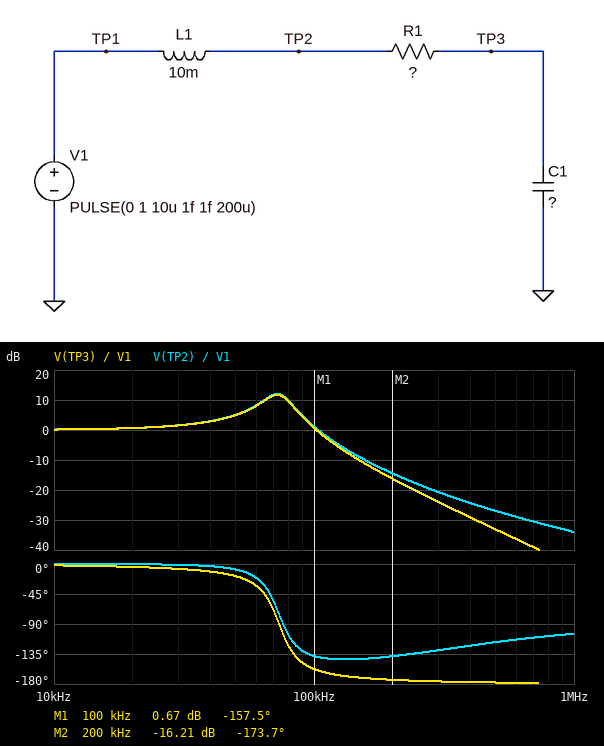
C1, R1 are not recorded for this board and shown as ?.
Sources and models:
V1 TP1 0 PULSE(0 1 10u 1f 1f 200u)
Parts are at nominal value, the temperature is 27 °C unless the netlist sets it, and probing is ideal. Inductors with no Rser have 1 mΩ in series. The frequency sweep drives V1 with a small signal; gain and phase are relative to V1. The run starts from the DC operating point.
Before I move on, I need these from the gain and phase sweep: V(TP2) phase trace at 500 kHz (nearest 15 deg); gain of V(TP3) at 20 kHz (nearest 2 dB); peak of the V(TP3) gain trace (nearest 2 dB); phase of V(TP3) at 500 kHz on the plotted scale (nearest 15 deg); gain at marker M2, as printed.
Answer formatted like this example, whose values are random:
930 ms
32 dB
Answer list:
-120 deg
0 dB
12 dB
-180 deg
-16.21 dB
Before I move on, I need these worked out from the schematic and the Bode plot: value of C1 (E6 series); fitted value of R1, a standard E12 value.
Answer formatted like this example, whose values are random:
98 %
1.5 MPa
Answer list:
470 pF
1.2 kΩ
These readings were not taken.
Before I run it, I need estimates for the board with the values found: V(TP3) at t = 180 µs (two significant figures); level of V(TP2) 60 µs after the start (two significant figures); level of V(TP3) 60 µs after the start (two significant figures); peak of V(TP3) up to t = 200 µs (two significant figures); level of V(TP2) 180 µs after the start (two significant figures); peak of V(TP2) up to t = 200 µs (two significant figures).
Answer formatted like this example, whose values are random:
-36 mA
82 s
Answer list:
1.0 V
1.0 V
1.0 V
1.7 V
1.0 V
1.7 V
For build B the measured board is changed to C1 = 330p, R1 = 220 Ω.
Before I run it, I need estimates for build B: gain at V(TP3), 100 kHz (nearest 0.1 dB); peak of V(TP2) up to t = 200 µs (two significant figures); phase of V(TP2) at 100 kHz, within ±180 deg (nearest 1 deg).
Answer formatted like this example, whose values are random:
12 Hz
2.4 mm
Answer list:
10.3 dB
1.9 V
-169 deg
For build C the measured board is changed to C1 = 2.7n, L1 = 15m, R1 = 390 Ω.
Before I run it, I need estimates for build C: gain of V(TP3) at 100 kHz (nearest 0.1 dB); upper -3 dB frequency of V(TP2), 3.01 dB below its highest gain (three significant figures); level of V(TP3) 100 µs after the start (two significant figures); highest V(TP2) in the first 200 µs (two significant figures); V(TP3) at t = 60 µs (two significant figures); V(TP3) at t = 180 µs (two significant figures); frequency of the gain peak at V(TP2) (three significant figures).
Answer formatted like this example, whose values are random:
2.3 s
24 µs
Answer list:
-23.5 dB
26.8 kHz
960 mV
1.8 V
940 mV
980 mV
24.8 kHz
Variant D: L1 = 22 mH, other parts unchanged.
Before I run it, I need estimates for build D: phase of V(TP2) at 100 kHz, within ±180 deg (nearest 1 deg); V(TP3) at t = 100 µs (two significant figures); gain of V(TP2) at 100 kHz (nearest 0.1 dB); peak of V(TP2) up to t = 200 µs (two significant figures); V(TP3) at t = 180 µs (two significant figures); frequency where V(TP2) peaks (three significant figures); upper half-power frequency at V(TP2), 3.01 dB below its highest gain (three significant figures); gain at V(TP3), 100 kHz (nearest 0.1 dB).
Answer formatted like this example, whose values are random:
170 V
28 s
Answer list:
-154 deg
1.1 V
-9.3 dB
1.8 V
1.0 V
49.1 kHz
53.3 kHz
-9.8 dB
